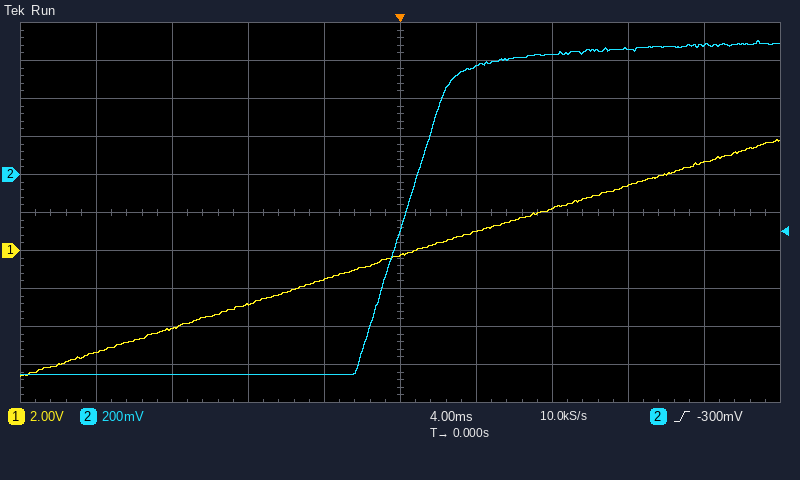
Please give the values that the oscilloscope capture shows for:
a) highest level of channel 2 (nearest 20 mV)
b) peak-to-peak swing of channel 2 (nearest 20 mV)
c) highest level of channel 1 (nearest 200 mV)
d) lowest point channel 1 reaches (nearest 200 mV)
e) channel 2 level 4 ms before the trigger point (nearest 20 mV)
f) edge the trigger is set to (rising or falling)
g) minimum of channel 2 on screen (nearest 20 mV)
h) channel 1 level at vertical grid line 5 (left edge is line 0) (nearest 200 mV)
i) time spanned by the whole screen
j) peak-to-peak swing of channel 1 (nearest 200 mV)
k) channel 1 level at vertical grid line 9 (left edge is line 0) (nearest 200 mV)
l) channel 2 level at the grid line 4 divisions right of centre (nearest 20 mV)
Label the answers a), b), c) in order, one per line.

a) 700 mV
b) 1.76 V
c) 5.8 V
d) -6.6 V
e) -1.06 V
f) rising
g) -1.06 V
h) -200 mV
i) 40 ms
j) 12.4 V
k) 4.6 V
l) 680 mV
